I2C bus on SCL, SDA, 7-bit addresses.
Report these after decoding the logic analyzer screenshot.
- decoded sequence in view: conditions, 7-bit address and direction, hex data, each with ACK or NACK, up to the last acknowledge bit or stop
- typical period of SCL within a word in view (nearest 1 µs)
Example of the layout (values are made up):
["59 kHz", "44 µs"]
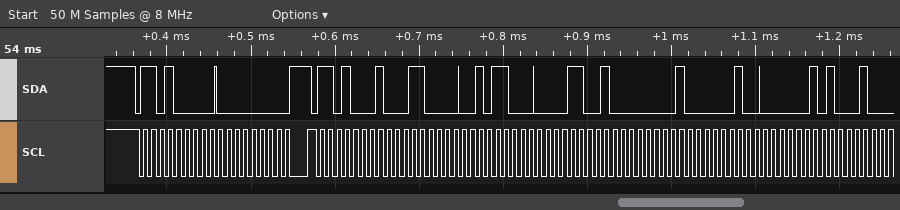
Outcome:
["start, address 68 write ACK, 00 ACK, repeated start, address 68 read ACK, 30 ACK, 58 ACK, 19 ACK, 01 ACK, 04 ACK, 05 ACK", "10 µs"]
